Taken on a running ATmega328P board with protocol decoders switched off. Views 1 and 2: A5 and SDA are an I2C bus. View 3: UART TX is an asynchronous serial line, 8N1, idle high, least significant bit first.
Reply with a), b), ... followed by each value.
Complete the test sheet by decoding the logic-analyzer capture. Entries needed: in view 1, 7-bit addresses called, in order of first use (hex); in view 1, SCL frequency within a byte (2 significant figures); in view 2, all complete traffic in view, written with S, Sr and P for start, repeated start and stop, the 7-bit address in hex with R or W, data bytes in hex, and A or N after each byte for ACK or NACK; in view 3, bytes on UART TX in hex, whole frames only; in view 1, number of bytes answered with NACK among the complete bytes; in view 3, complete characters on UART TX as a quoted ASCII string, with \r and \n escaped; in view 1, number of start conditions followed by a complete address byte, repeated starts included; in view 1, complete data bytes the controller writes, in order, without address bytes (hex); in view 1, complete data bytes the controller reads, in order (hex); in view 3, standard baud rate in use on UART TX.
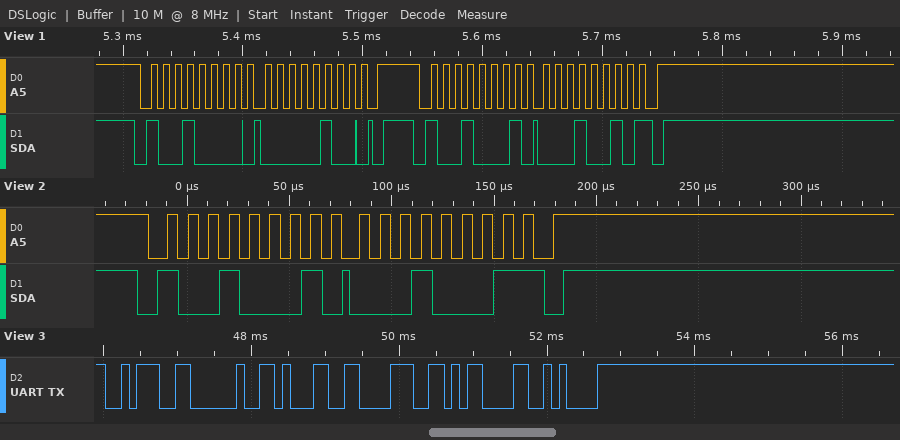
a) 0x48
b) 100 kHz
c) S 48R A 11 N P
d) 3A 20 31 38 0D 0A
e) 1
f) ": 18\r\n"
g) 2
h) 04
i) 12
j) 9600 baud
